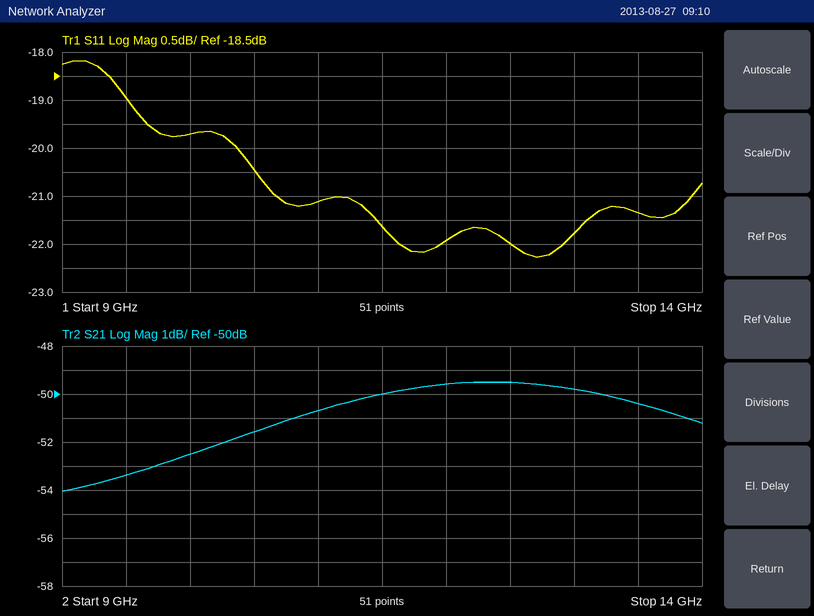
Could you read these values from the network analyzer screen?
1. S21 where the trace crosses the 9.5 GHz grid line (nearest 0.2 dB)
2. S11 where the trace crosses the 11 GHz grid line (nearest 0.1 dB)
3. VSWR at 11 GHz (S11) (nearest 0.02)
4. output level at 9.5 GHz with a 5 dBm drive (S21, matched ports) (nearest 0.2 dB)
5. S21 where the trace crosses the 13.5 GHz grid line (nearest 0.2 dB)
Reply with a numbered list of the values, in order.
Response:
1. -53.4 dB
2. -21.1 dB
3. 1.20
4. -48.4 dBm
5. -50.4 dB
